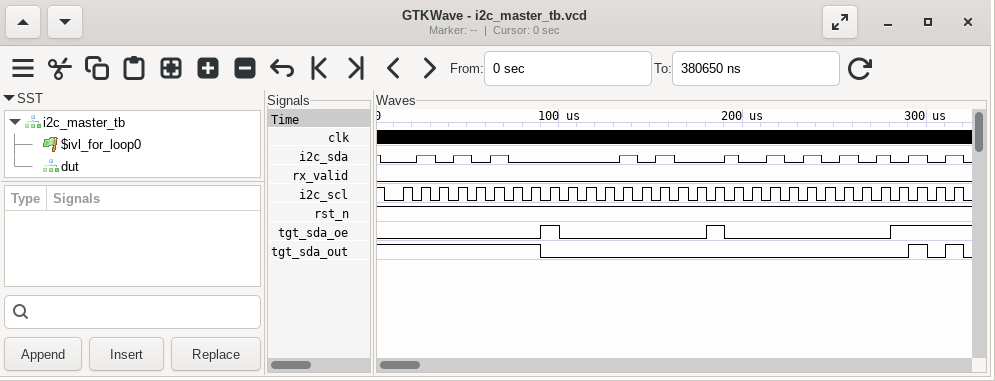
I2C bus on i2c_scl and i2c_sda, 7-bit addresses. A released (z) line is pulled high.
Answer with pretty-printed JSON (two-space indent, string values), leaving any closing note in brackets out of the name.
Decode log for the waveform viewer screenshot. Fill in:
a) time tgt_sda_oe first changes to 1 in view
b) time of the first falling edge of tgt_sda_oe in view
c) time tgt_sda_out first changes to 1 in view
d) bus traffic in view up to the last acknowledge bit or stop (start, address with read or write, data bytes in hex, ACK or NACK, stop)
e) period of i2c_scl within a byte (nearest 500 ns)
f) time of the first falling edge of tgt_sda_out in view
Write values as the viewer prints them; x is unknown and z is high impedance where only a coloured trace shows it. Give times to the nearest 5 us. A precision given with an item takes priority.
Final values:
{
  "time tgt_sda_oe first changes to 1 in view": "90 us",
  "time of the first falling edge of tgt_sda_oe in view": "100 us",
  "time tgt_sda_out first changes to 1 in view": "290 us",
  "bus traffic in view up to the last acknowledge bit or stop": "start, address 2A write ACK, 14 ACK, repeated start, address 2A read ACK",
  "period of i2c_scl within a byte": "10000 ns",
  "time of the first falling edge of tgt_sda_out in view": "90 us"
}
